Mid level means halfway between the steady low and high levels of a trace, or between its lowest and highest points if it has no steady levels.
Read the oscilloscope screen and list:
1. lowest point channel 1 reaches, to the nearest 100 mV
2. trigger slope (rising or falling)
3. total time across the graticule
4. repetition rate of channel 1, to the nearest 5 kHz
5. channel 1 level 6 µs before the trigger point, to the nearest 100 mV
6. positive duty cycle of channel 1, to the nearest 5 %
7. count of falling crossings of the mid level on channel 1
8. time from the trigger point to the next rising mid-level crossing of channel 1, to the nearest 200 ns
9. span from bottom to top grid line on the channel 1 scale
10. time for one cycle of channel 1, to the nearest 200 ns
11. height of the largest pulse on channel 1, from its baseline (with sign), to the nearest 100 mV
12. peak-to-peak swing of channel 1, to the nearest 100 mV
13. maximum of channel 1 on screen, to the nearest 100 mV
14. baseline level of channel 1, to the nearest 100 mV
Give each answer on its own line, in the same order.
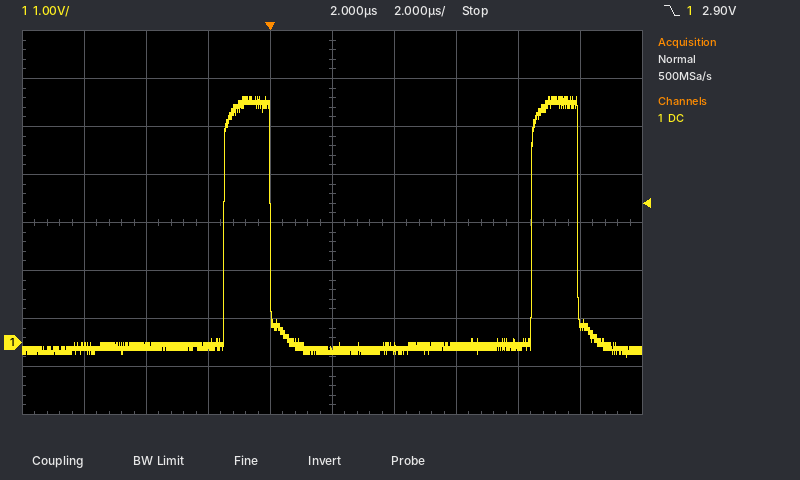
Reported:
-300 mV
falling
20 µs
100 kHz
-100 mV
15 %
2
8.4 µs
8 V
10.0 µs
+5.2 V
5.4 V
5.1 V
-100 mV
